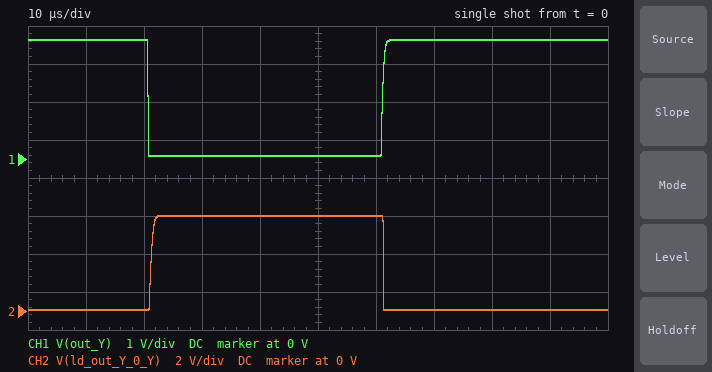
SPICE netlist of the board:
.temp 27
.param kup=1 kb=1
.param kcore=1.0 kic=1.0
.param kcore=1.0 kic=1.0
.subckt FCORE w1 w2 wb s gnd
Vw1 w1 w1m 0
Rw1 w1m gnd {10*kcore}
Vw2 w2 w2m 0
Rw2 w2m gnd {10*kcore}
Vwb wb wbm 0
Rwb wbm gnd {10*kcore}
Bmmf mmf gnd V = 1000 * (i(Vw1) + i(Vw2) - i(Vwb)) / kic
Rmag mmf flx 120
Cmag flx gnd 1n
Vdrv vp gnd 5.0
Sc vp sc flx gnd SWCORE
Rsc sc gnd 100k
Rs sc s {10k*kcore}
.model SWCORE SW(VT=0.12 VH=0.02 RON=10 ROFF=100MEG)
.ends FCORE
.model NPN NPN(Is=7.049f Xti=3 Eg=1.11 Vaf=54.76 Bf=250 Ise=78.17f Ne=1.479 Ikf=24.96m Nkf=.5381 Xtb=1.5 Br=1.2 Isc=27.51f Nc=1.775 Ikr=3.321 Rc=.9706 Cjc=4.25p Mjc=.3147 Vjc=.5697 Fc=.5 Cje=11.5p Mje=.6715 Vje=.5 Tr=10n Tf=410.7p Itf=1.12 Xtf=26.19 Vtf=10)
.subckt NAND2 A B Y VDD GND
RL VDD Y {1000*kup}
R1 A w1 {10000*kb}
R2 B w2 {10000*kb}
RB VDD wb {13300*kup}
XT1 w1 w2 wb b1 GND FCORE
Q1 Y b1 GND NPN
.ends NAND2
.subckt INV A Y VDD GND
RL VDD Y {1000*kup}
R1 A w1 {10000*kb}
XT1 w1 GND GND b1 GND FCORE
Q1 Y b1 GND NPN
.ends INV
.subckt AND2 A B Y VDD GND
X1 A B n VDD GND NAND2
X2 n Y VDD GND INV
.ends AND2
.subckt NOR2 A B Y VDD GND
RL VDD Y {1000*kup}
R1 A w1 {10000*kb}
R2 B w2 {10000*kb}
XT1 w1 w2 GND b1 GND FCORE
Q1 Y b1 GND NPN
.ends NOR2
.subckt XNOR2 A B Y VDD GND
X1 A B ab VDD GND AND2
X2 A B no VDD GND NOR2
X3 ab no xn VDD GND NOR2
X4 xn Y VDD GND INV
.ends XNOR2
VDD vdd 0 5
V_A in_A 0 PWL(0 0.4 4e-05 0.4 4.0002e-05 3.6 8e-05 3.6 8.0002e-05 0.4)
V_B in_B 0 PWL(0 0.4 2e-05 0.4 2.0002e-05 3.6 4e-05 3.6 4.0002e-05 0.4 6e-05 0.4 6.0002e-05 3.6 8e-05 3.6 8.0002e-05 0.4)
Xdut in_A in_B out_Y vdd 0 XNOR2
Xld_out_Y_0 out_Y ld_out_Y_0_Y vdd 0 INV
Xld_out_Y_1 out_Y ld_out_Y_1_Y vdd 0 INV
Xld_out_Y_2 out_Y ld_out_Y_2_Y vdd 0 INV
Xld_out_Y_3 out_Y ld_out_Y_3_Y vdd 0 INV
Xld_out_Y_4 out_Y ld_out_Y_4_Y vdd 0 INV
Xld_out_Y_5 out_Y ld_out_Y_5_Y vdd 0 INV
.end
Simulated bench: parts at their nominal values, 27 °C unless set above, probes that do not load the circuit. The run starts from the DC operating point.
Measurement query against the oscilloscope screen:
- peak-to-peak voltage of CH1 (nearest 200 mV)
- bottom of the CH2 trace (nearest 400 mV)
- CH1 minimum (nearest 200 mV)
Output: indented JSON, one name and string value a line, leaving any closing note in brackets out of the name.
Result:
{
  "peak-to-peak voltage of CH1": "3.0 V",
  "bottom of the CH2 trace": "0 V",
  "CH1 minimum": "0 V"
}
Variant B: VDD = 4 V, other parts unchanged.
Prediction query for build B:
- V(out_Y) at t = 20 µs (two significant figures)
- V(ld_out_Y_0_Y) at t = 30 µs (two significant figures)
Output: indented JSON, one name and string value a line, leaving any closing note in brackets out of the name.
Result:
{
  "V(out_Y) at t = 20 µs": "2.5 V",
  "V(ld_out_Y_0_Y) at t = 30 µs": "4.0 V"
}
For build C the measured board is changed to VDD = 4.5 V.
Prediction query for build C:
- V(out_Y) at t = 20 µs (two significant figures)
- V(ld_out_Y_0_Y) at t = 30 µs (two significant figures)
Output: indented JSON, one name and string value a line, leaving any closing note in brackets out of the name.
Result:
{
  "V(out_Y) at t = 20 µs": "2.8 V",
  "V(ld_out_Y_0_Y) at t = 30 µs": "4.5 V"
}
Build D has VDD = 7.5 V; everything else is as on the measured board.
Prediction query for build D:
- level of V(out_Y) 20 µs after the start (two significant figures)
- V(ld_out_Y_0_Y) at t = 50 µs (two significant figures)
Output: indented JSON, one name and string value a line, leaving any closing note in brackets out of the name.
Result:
{
  "level of V(out_Y) 20 µs after the start": "4.7 V",
  "V(ld_out_Y_0_Y) at t = 50 µs": "7.5 V"
}
